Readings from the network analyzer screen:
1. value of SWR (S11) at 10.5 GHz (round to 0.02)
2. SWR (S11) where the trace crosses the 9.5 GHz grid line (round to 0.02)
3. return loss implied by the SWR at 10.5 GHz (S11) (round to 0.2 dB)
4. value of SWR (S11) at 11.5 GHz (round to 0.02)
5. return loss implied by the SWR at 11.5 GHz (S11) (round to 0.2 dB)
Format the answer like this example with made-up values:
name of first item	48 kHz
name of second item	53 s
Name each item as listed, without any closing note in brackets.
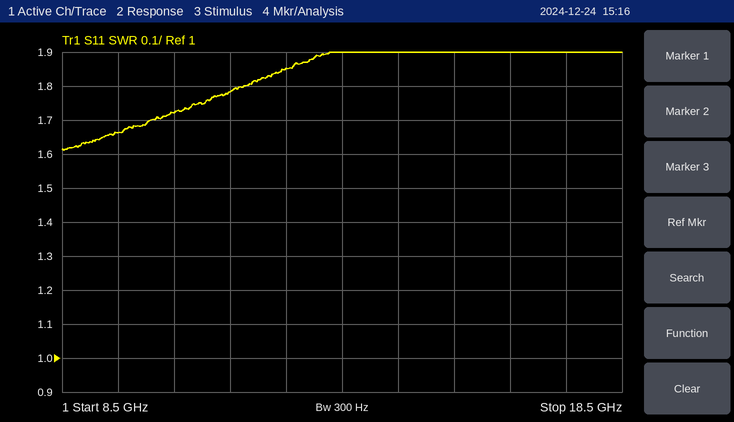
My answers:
value of SWR (S11) at 10.5 GHz	1.72
SWR (S11) where the trace crosses the 9.5 GHz grid line	1.66
return loss implied by the SWR at 10.5 GHz (S11)	11.6 dB
value of SWR (S11) at 11.5 GHz	1.78
return loss implied by the SWR at 11.5 GHz (S11)	11.0 dB
